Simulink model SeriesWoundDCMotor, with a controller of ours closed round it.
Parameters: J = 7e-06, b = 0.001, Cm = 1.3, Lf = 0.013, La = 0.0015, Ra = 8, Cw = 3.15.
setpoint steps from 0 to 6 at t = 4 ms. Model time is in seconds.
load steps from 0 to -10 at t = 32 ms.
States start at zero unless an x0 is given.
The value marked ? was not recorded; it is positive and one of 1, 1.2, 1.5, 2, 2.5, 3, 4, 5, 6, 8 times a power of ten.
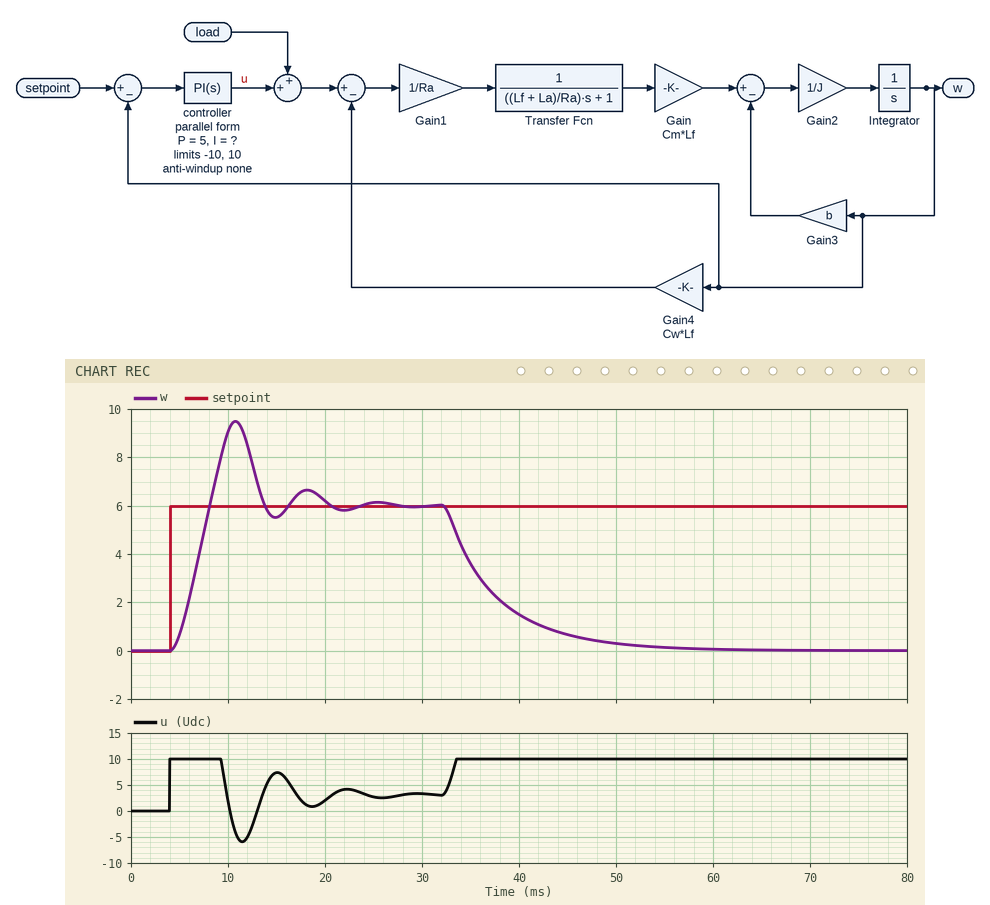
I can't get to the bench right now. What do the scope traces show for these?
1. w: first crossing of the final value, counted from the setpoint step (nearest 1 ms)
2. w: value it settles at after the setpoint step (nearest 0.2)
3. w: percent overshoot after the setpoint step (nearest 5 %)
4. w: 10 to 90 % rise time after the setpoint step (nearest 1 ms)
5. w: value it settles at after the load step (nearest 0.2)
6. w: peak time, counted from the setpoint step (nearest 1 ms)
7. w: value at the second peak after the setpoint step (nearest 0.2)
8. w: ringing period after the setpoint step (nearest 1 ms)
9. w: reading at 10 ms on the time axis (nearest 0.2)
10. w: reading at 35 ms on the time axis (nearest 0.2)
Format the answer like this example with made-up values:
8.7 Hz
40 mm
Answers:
4 ms
6.0
60 %
3 ms
0.0
7 ms
6.6
7 ms
9.0
3.6
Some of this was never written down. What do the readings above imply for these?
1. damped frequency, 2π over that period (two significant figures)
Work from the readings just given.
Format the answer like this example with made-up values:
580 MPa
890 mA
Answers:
0.90 rad/ms
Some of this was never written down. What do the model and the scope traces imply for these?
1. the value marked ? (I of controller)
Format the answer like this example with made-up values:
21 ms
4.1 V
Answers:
1500
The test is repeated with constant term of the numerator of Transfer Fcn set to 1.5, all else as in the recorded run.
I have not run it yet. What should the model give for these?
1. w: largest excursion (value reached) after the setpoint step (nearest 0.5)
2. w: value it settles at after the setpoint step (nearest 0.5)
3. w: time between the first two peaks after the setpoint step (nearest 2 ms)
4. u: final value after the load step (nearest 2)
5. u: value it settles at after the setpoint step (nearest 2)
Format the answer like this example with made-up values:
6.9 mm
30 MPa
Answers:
9.5
6.0
6 ms
10
2
